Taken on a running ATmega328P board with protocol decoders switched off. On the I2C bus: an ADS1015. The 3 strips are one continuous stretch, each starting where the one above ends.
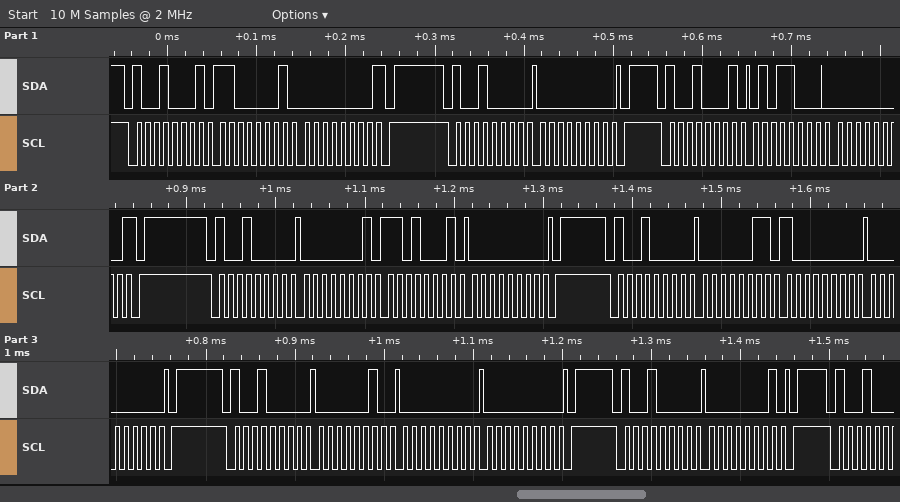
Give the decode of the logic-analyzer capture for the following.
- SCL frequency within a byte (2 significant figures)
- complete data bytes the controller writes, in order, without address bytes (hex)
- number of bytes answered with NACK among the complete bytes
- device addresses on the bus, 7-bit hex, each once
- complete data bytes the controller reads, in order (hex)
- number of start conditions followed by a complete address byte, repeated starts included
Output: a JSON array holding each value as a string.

["100 kHz", "00 01 D1 00 03 80 00 02 00 00 01", "2", "0x48", "C1 00 58 00", "7"]
